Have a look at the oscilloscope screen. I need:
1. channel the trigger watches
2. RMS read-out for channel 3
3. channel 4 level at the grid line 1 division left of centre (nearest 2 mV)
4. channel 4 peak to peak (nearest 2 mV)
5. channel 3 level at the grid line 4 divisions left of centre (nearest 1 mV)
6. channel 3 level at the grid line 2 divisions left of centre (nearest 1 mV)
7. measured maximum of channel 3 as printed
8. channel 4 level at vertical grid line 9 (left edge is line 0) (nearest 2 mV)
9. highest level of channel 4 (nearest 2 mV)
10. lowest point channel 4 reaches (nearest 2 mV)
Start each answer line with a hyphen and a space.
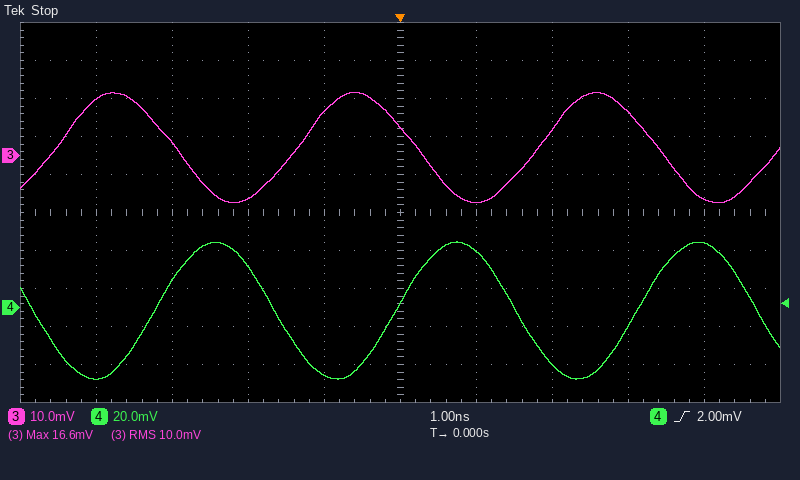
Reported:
- channel 4
- 10.0 mV
- -36 mV
- 72 mV
- 15 mV
- -11 mV
- 16.6 mV
- 34 mV
- 34 mV
- -38 mV
